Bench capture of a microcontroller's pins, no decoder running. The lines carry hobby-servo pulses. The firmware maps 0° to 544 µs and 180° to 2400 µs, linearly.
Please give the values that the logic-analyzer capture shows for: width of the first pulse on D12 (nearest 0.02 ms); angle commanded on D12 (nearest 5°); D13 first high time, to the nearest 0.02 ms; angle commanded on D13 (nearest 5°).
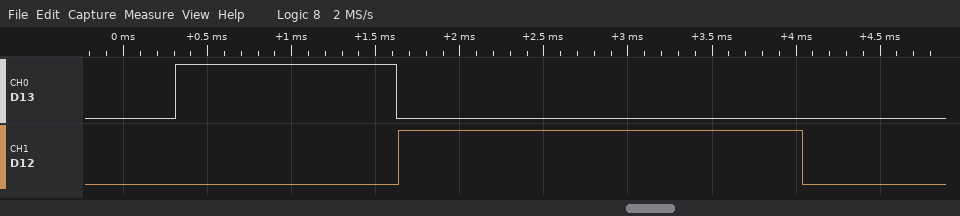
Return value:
2.40 ms
180°
1.32 ms
75°
